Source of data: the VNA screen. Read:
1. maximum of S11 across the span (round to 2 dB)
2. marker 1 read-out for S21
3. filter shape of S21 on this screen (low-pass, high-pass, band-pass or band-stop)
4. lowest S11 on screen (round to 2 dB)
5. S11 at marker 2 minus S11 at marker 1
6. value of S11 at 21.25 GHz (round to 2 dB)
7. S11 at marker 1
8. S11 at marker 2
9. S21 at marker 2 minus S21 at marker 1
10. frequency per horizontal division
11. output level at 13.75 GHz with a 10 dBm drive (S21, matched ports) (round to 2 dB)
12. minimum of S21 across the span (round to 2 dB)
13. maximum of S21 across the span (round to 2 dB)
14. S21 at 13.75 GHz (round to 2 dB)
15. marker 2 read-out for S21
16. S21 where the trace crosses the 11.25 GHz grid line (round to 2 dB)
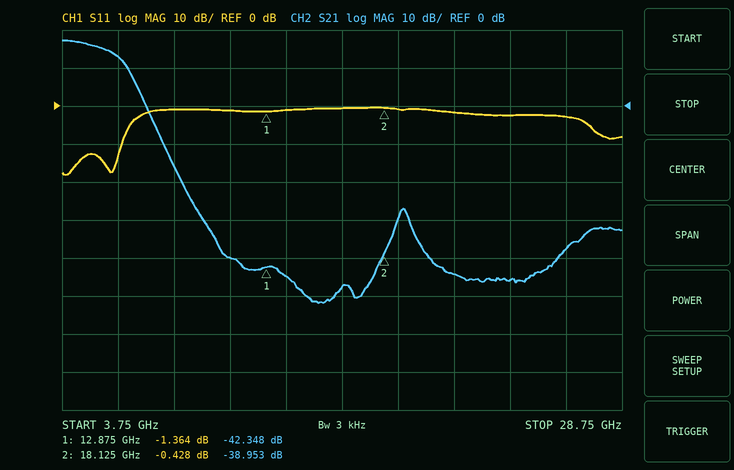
0 dB
-42.348 dB
low-pass
-18 dB
0.936 dB
-2 dB
-1.364 dB
-0.428 dB
3.395 dB
2.5 GHz
-34 dBm
-52 dB
18 dB
-44 dB
-38.953 dB
-40 dB
